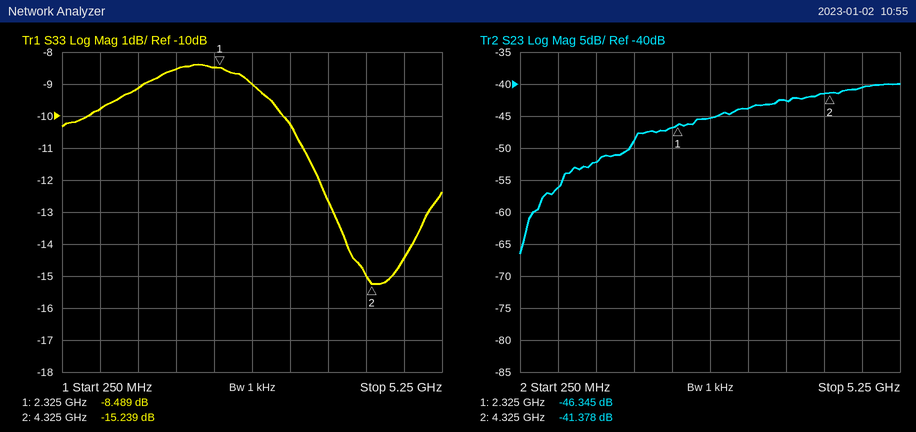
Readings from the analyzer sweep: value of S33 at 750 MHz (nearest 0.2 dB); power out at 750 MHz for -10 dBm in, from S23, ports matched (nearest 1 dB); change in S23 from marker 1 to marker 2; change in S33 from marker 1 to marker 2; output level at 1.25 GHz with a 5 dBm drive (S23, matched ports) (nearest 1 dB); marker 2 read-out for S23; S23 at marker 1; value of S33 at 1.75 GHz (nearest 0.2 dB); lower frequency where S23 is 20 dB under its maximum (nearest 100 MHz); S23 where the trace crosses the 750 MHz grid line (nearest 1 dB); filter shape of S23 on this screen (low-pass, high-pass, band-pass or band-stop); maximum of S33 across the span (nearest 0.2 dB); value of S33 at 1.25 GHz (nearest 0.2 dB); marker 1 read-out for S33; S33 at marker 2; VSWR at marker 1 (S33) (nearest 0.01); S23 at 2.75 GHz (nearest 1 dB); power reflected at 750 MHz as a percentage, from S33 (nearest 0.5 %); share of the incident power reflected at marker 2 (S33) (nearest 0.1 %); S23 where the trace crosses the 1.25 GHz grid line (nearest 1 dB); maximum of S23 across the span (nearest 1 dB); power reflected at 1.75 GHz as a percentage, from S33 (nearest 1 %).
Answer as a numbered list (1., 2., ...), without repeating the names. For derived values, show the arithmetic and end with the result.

1. -9.8 dB
2. -10 dBm + (-56 dB) = -66 dBm
3. -41.378 − (-46.345) = 4.967 dB
4. -15.239 − (-8.489) = -6.750 dB
5. 5 dBm + (-52 dB) = -47 dBm
6. -41.378 dB
7. -46.345 dB
8. -8.6 dB
9. 400 MHz
10. -56 dB
11. high-pass
12. -8.4 dB
13. -9.2 dB
14. -8.489 dB
15. -15.239 dB
16. (1 + 0.3763)/(1 − 0.3763) ≈ 2.21
17. -45 dB
18. 10^(-9.8/10) ≈ 10.5 %
19. 10^(-15.239/10) ≈ 3.0 %
20. -52 dB
21. -40 dB
22. 10^(-8.6/10) ≈ 14 %
